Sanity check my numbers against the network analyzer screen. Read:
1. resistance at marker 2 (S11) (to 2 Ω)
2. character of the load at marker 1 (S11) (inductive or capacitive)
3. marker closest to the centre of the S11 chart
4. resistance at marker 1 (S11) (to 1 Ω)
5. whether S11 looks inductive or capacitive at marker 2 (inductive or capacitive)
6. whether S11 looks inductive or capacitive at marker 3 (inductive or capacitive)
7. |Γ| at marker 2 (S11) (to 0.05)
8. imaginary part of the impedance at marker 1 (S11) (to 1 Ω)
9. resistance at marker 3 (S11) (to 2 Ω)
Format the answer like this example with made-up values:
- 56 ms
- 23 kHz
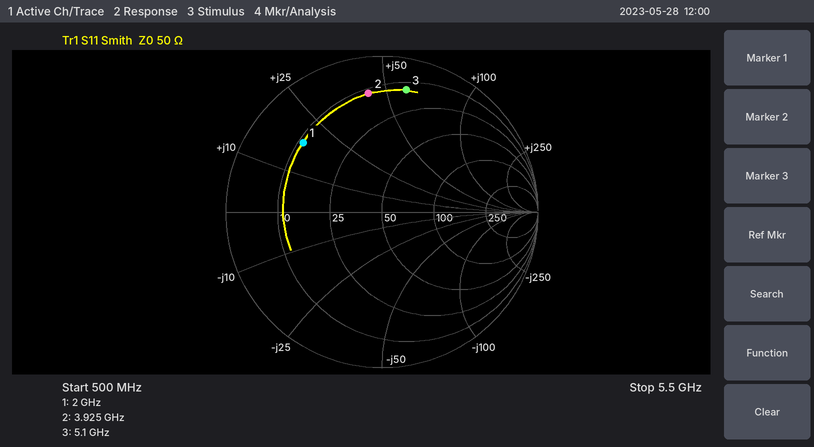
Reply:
- 12 Ω
- inductive
- marker 1
- 11 Ω
- inductive
- inductive
- 0.75
- +18 Ω
- 14 Ω
